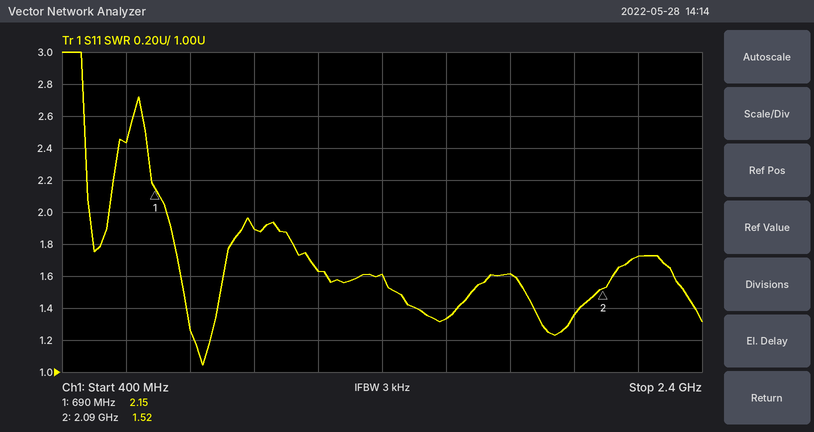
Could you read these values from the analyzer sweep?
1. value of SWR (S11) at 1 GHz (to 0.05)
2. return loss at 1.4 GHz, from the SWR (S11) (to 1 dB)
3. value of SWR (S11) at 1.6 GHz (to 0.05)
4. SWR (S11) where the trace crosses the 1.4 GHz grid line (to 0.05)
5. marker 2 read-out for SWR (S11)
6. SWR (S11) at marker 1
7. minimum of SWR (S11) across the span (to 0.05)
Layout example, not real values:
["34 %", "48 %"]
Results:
["1.90", "13 dB", "1.35", "1.60", "1.52", "2.15", "1.05"]
